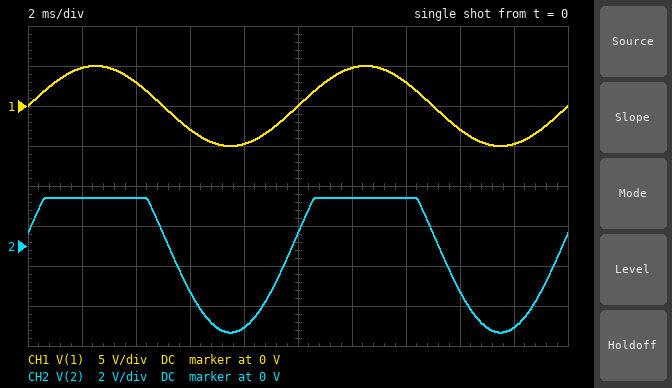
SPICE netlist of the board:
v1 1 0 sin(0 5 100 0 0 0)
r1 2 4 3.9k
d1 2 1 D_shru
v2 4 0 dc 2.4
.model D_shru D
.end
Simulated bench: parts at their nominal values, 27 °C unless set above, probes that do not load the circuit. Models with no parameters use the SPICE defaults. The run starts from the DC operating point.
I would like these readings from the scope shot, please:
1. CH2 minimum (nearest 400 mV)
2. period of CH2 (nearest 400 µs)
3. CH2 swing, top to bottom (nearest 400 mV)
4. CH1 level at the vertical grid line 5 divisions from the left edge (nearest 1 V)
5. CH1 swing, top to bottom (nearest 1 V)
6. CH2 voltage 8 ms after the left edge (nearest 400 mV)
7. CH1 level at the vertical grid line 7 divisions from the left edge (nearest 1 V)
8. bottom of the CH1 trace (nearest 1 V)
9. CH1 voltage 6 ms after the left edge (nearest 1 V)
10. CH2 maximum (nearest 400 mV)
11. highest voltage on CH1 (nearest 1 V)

-4.4 V
10.0 ms
6.8 V
0 V
10 V
-4.0 V
3 V
-5 V
-3 V
2.4 V
5 V
